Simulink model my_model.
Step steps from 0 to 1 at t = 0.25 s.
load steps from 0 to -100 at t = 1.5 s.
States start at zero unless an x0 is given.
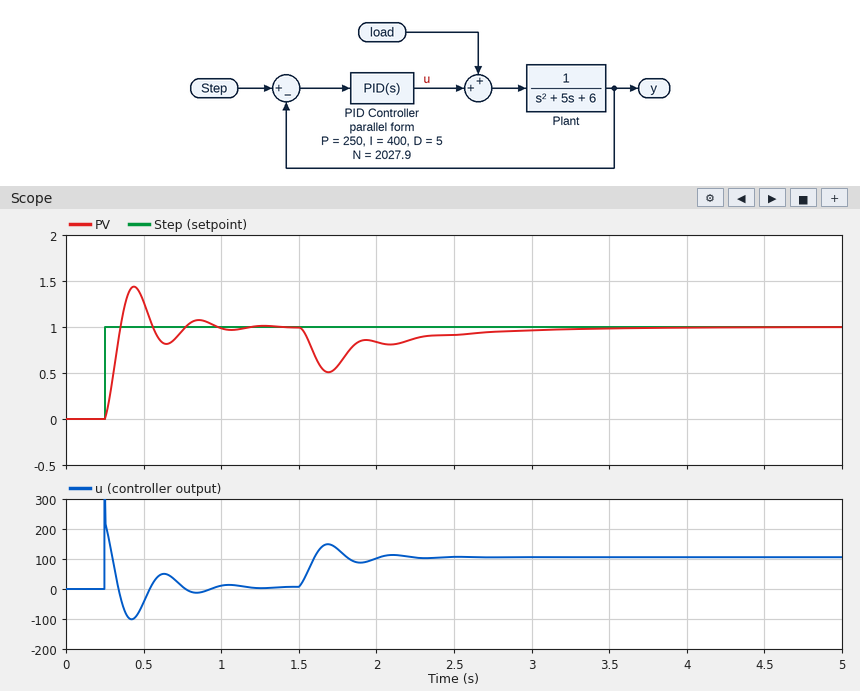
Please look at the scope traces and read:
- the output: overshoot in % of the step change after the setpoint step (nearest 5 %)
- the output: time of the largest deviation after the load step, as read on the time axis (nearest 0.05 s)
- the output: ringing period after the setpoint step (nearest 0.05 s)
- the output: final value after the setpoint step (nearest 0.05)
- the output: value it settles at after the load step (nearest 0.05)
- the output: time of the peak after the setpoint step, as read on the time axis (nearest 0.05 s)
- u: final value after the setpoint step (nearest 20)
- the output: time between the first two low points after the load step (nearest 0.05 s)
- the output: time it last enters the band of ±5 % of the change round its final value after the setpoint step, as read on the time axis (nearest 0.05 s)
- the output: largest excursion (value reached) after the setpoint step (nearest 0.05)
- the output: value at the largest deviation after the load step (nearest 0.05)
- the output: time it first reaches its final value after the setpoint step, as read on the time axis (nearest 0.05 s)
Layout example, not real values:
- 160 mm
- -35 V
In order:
- 45 %
- 1.70 s
- 0.40 s
- 1.00
- 1.00
- 0.45 s
- 0
- 0.40 s
- 0.90 s
- 1.45
- 0.50
- 0.35 s
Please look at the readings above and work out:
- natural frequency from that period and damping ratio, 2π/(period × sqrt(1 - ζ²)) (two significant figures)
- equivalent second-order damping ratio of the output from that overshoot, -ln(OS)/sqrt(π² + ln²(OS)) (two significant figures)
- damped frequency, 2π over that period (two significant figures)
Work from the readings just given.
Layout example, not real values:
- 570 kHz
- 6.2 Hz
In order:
- 16 rad/s
- 0.25
- 16 rad/s
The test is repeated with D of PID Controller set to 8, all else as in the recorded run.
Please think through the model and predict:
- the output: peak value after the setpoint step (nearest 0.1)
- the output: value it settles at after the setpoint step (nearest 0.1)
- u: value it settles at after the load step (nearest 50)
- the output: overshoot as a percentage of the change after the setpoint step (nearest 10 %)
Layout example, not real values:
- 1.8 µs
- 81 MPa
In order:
- 1.3
- 1.0
- 100
- 30 %
